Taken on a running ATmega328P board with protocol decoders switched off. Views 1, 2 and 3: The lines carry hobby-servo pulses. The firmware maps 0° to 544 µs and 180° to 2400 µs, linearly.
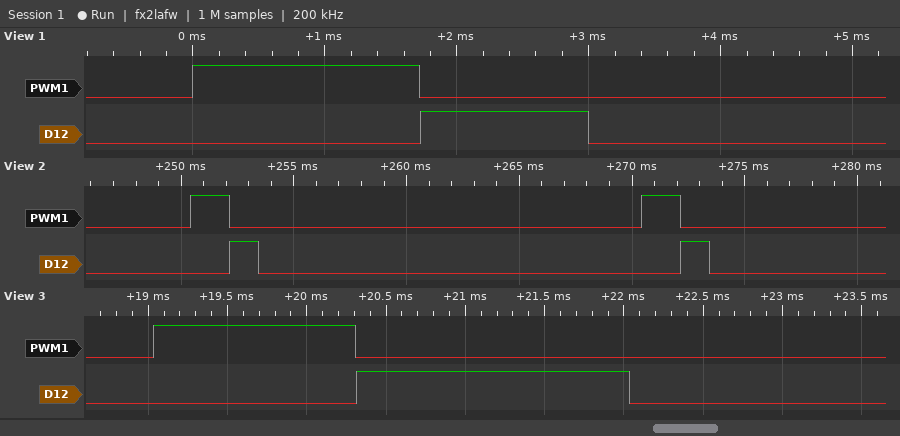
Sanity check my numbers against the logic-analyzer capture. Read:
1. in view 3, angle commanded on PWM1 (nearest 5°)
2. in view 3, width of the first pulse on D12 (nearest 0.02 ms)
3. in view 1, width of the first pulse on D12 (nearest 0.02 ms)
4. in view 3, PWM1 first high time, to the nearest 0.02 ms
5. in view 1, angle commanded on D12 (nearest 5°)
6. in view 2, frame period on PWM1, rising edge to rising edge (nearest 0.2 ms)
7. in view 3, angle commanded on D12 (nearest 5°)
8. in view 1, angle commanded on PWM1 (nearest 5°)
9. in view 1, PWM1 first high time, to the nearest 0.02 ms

70°
1.72 ms
1.28 ms
1.28 ms
70°
20.0 ms
115°
115°
1.72 ms
